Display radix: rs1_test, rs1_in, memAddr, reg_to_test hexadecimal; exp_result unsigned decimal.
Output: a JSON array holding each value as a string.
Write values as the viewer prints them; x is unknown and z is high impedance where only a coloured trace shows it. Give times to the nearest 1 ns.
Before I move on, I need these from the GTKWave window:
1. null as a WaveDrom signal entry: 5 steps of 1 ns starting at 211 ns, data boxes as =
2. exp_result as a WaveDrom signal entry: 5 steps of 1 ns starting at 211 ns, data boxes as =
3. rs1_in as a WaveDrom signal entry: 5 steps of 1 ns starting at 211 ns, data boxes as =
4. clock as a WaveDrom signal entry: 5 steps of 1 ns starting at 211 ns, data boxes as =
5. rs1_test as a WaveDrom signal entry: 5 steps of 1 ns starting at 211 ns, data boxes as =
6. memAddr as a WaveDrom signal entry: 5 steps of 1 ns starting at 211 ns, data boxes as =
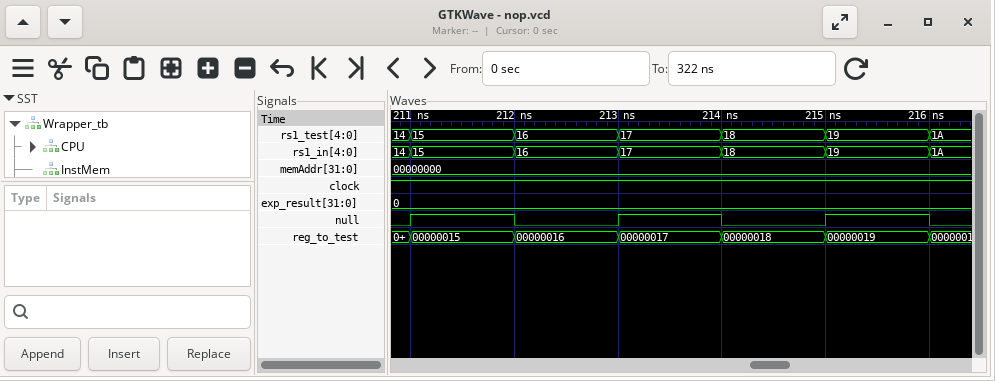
["{name: 'null', wave: '10101'}", "{name: 'exp_result', wave: '=....', data: '0'}", "{name: 'rs1_in', wave: '=====', data: '15 16 17 18 19'}", "{name: 'clock', wave: '1....'}", "{name: 'rs1_test', wave: '=====', data: '15 16 17 18 19'}", "{name: 'memAddr', wave: '=....', data: '00000000'}"]
